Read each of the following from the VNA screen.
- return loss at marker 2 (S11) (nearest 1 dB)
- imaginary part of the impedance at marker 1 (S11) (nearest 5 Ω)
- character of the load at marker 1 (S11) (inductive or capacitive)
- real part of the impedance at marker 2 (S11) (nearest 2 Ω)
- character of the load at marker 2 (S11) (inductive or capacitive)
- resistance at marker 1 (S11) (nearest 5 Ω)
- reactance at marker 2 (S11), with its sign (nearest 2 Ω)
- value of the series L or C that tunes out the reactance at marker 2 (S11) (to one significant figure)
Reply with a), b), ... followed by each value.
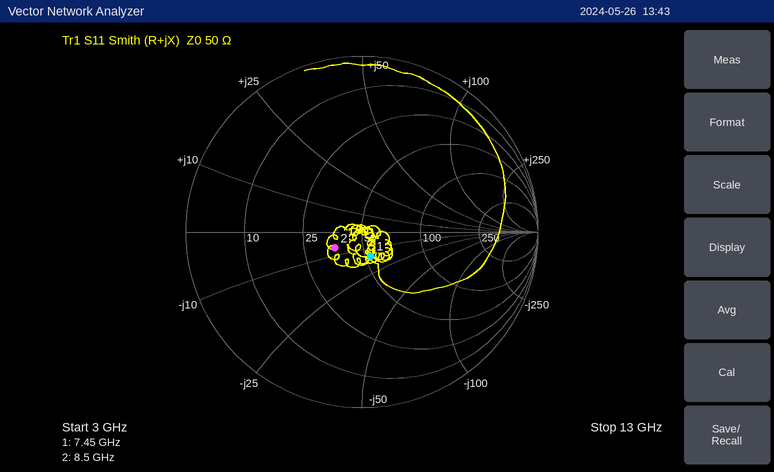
a) 15 dB
b) -15 Ω
c) capacitive
d) 36 Ω
e) capacitive
f) 55 Ω
g) -6 Ω
h) 100 pH
